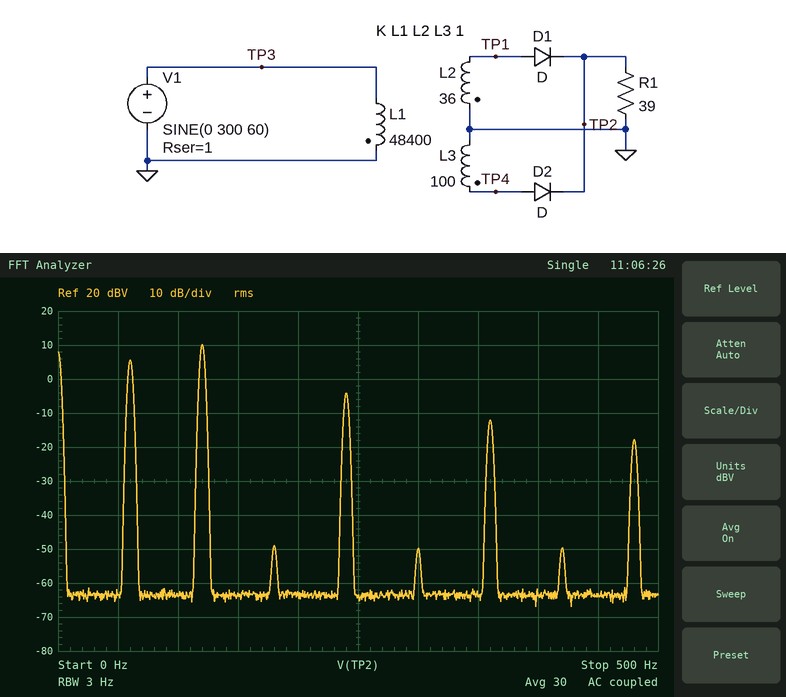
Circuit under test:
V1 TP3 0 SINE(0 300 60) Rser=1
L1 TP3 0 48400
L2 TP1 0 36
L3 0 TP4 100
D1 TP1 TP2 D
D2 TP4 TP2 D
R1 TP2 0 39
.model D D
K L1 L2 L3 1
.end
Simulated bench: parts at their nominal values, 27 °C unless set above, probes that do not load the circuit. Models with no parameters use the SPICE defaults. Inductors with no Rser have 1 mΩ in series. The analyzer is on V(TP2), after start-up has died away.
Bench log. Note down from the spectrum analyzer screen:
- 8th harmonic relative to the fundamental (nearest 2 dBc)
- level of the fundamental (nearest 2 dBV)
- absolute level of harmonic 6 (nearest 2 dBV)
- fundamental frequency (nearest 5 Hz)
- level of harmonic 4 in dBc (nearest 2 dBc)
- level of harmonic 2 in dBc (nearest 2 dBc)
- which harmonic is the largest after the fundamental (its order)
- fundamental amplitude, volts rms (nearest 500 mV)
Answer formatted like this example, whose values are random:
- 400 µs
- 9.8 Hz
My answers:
- -24 dBc
- 6 dBV
- -12 dBV
- 60 Hz
- -10 dBc
- 4 dBc
- 2
- 2.0 V
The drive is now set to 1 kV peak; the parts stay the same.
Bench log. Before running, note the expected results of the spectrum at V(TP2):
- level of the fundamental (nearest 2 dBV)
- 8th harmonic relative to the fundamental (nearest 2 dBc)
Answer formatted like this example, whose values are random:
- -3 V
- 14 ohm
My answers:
- 16 dBV
- -22 dBc
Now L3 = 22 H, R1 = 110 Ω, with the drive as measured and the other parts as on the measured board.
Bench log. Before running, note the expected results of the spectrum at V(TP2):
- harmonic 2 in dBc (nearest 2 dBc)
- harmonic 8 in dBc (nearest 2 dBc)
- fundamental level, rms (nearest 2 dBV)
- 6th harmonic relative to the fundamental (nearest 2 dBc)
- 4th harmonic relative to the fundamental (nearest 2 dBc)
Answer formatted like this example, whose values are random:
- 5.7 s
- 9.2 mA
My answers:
- 10 dBc
- -18 dBc
- -4 dBV
- -12 dBc
- -4 dBc
